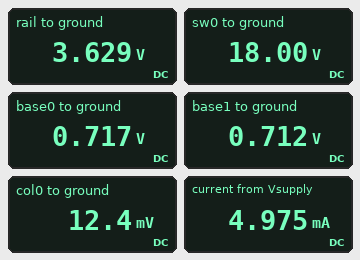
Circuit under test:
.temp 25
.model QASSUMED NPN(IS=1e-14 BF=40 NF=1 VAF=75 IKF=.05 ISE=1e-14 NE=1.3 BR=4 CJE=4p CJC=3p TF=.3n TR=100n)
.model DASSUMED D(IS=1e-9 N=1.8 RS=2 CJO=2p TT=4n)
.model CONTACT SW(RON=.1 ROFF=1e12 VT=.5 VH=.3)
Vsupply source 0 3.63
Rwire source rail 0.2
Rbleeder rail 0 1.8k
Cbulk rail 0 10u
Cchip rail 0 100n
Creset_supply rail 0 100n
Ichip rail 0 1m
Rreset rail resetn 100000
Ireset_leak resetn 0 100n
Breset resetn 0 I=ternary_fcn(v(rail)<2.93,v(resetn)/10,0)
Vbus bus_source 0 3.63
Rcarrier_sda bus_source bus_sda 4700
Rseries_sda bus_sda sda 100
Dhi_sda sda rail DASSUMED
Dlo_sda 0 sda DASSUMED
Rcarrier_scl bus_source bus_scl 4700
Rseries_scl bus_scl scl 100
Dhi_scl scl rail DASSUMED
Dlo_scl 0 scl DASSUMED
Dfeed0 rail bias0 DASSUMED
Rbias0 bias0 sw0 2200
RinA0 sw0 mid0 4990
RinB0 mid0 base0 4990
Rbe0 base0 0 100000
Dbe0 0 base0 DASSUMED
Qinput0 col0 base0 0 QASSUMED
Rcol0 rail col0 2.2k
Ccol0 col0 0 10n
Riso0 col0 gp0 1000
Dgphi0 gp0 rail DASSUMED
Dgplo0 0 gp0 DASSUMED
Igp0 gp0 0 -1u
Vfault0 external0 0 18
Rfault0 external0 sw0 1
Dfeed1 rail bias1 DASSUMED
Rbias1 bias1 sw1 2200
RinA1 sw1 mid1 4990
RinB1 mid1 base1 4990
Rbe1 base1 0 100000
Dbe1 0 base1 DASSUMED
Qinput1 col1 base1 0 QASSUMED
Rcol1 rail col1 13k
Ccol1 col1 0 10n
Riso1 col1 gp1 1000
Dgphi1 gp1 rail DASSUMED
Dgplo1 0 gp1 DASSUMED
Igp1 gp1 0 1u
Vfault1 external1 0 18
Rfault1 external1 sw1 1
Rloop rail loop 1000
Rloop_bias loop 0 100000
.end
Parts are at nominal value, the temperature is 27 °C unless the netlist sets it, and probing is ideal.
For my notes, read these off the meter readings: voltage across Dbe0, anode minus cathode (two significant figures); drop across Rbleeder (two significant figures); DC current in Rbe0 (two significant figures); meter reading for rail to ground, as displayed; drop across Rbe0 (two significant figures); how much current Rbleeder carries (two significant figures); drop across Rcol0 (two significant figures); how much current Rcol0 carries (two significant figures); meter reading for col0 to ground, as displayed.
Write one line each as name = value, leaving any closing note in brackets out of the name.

voltage across Dbe0, anode minus cathode = -720 mV
drop across Rbleeder = 3.6 V
DC current in Rbe0 = 7.2 µA
meter reading for rail to ground, as displayed = 3.629 V
drop across Rbe0 = 720 mV
how much current Rbleeder carries = 2.0 mA
drop across Rcol0 = 3.6 V
how much current Rcol0 carries = 1.6 mA
meter reading for col0 to ground, as displayed = 12.4 mV
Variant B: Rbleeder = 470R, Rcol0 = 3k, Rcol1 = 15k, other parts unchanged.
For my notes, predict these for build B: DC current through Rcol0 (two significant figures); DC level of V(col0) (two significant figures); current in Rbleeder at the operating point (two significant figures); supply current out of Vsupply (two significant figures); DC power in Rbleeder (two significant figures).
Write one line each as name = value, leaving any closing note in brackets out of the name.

DC current through Rcol0 = 1.2 mA
DC level of V(col0) = 11 mV
current in Rbleeder at the operating point = 7.7 mA
supply current out of Vsupply = 10 mA
DC power in Rbleeder = 28 mW
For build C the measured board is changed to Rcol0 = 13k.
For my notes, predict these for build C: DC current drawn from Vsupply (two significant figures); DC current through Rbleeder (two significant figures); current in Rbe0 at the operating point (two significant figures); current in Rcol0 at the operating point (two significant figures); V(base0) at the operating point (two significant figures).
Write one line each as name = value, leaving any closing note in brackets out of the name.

DC current drawn from Vsupply = 3.6 mA
DC current through Rbleeder = 2.0 mA
current in Rbe0 at the operating point = 7.1 µA
current in Rcol0 at the operating point = 280 µA
V(base0) at the operating point = 710 mV
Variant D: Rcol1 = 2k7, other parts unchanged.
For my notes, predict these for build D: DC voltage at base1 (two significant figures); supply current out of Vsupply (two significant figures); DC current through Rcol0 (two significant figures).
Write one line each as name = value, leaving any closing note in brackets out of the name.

DC voltage at base1 = 720 mV
supply current out of Vsupply = 6.0 mA
DC current through Rcol0 = 1.6 mA
